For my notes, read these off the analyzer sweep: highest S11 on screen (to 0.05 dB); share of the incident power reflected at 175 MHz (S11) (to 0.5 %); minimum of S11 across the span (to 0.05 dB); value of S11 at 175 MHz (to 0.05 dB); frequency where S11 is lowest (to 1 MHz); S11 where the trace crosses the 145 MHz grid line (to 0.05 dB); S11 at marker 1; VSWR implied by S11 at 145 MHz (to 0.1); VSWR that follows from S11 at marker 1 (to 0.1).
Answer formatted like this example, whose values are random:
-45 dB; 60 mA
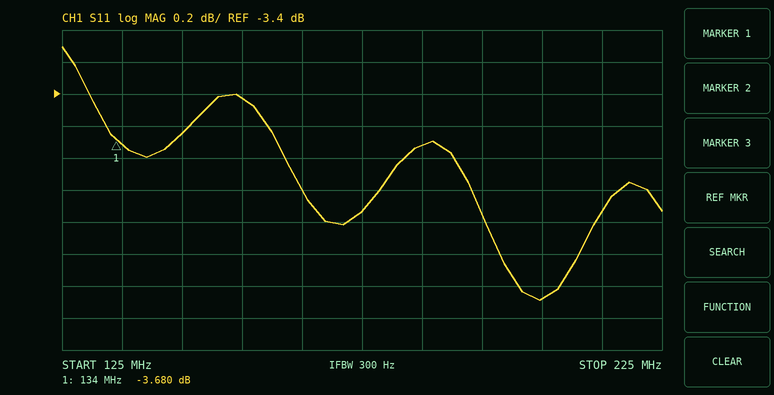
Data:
-3.10 dB; 38.5 %; -4.70 dB; -4.15 dB; 205 MHz; -3.65 dB; -3.680 dB; 4.8; 4.8
